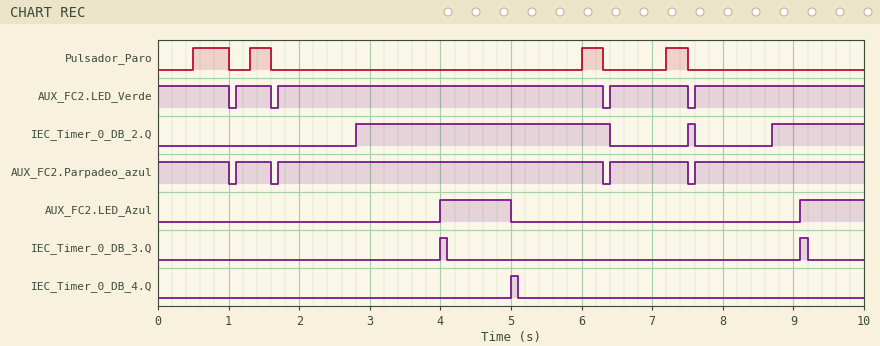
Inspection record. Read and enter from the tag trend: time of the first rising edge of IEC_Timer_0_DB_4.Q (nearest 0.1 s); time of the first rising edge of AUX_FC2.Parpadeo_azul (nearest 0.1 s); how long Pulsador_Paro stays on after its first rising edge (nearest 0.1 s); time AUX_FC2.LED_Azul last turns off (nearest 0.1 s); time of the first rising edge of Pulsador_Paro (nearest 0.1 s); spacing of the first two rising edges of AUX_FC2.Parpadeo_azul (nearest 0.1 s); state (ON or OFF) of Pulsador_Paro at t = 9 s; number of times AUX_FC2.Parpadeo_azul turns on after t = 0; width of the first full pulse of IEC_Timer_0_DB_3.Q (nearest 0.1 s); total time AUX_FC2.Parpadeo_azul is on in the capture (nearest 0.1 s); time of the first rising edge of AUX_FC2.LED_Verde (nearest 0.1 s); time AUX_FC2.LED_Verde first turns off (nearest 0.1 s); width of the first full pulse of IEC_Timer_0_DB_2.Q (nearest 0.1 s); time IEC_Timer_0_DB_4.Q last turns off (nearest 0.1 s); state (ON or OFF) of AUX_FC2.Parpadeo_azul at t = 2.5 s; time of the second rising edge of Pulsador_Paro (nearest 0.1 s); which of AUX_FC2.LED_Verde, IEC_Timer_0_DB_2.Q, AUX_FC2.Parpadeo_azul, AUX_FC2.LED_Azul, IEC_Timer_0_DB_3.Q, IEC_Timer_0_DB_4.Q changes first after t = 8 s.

5.0 s
1.1 s
0.5 s
5.0 s
0.5 s
0.6 s
OFF
4
0.1 s
9.6 s
1.1 s
1.0 s
3.6 s
5.1 s
ON
1.3 s
IEC_Timer_0_DB_2.Q
